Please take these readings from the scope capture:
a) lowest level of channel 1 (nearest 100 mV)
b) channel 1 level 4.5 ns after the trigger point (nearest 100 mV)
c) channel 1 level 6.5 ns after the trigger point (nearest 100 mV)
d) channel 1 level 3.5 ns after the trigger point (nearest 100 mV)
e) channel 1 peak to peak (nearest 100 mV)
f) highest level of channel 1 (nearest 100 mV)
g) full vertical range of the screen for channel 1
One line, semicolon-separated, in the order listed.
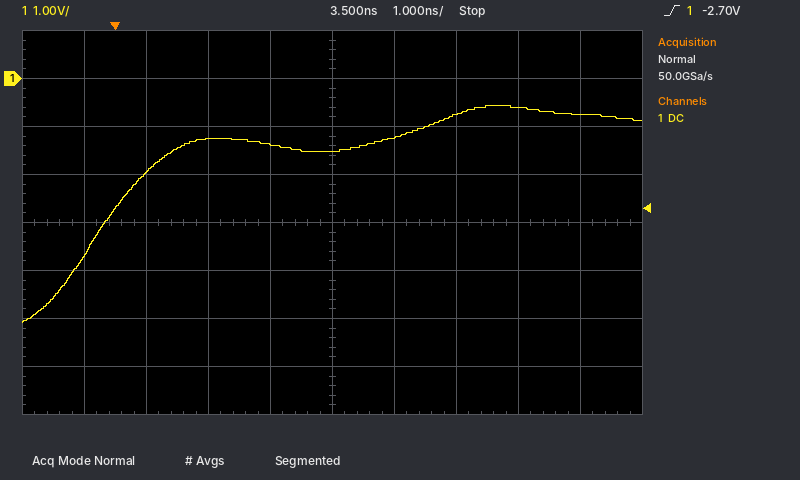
-5.1 V; -1.2 V; -600 mV; -1.5 V; 4.5 V; -600 mV; 8 V
